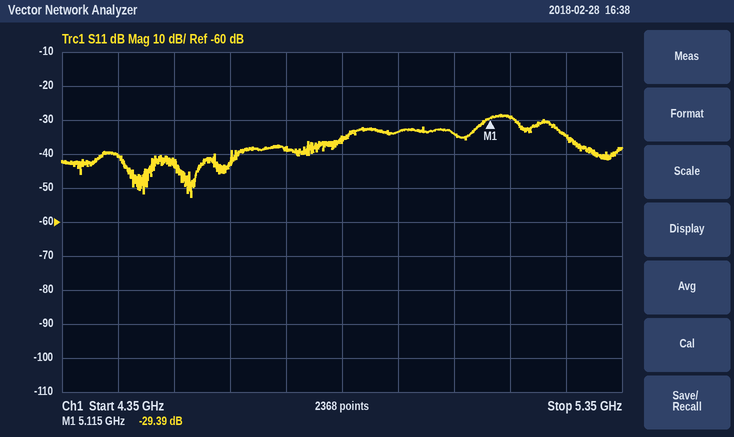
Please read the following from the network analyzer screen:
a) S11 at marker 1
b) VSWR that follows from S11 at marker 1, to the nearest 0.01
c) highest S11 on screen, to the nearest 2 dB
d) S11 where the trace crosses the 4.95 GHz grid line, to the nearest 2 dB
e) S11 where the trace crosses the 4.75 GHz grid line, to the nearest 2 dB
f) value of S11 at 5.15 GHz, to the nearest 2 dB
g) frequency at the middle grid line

-29.39 dB
1.07
-28 dB
-34 dB
-38 dB
-30 dB
4.85 GHz
